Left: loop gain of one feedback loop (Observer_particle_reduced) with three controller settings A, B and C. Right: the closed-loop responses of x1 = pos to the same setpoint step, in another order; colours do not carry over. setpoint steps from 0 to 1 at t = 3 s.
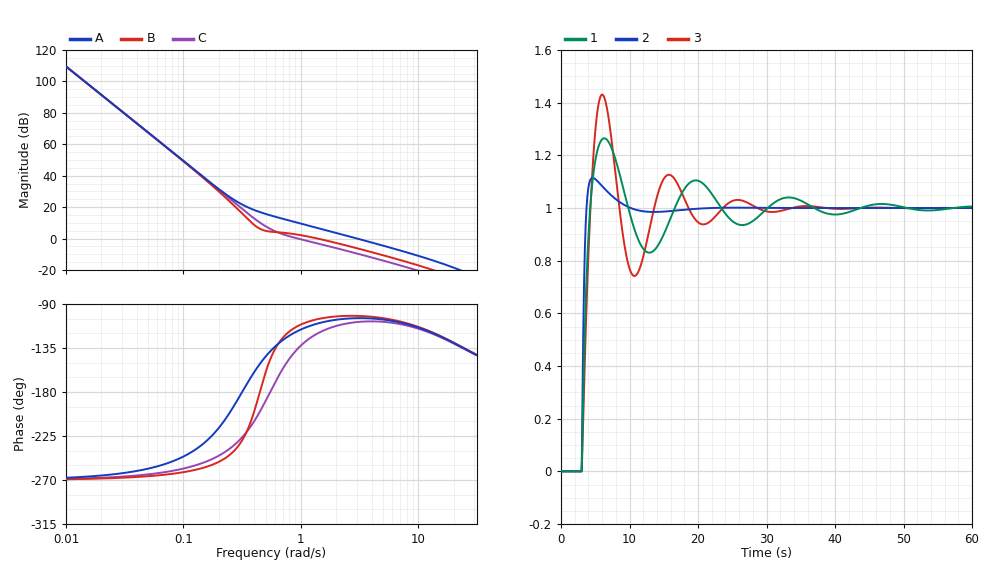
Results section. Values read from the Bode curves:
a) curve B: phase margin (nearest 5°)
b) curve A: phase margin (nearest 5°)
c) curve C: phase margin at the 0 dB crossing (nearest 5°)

75°
75°
45°
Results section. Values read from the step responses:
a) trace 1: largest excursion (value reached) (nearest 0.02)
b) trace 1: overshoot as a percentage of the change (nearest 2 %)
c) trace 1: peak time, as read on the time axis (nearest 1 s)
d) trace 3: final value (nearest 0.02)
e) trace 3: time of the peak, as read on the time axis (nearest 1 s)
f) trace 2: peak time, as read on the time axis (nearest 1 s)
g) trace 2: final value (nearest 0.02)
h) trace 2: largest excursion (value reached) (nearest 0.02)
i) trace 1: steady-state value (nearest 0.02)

1.26
26 %
6 s
1.00
6 s
5 s
1.00
1.12
1.00
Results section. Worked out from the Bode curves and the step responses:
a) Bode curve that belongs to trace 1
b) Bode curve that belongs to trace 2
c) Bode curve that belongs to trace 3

B
A
C
